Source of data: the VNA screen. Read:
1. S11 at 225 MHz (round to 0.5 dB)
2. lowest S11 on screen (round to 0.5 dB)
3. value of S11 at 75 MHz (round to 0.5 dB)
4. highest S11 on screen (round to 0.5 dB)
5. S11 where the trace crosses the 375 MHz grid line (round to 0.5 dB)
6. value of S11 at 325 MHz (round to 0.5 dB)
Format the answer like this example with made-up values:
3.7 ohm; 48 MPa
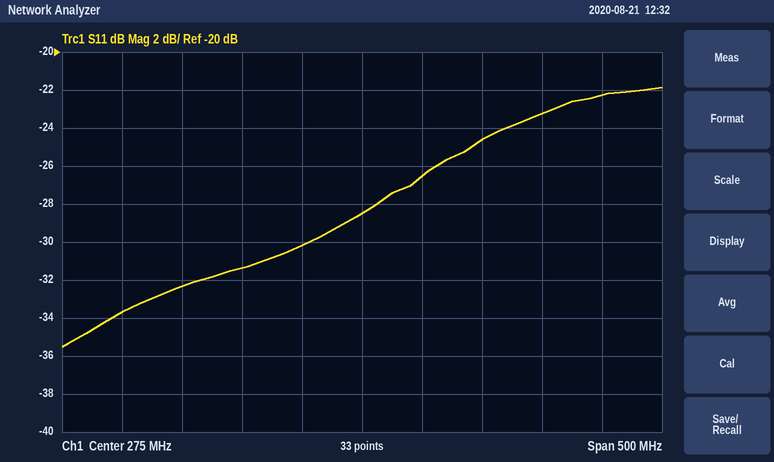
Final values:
-30.0 dB; -35.5 dB; -33.5 dB; -22.0 dB; -24.5 dB; -26.5 dB
